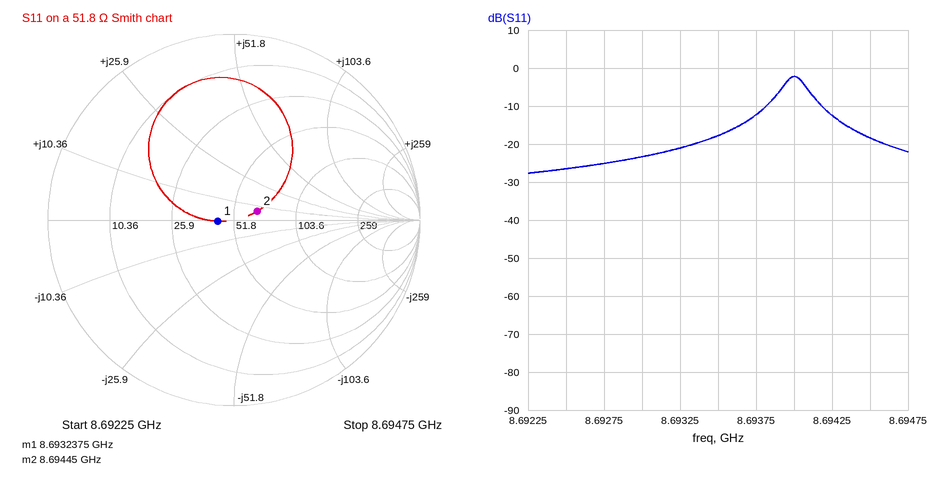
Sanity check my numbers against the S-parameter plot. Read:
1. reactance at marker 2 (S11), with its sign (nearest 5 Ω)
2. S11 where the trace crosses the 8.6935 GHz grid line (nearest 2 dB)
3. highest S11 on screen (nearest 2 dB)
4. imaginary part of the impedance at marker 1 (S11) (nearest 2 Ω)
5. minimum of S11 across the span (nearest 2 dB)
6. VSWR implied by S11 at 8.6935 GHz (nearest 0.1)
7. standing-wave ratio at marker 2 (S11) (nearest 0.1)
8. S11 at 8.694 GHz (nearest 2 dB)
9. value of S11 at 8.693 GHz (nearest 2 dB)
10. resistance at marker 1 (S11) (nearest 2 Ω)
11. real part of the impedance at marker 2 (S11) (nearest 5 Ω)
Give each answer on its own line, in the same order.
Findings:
+5 Ω
-18 dB
-2 dB
0 Ω
-28 dB
1.3
1.3
-2 dB
-24 dB
44 Ω
65 Ω
